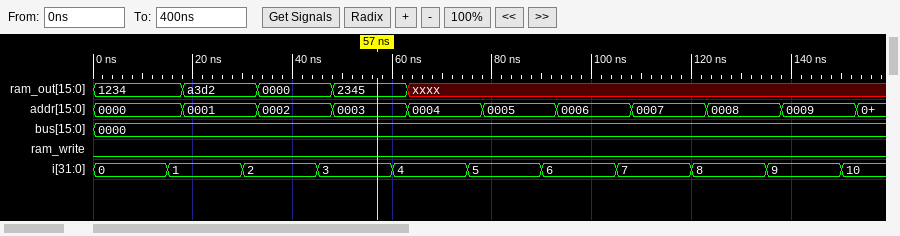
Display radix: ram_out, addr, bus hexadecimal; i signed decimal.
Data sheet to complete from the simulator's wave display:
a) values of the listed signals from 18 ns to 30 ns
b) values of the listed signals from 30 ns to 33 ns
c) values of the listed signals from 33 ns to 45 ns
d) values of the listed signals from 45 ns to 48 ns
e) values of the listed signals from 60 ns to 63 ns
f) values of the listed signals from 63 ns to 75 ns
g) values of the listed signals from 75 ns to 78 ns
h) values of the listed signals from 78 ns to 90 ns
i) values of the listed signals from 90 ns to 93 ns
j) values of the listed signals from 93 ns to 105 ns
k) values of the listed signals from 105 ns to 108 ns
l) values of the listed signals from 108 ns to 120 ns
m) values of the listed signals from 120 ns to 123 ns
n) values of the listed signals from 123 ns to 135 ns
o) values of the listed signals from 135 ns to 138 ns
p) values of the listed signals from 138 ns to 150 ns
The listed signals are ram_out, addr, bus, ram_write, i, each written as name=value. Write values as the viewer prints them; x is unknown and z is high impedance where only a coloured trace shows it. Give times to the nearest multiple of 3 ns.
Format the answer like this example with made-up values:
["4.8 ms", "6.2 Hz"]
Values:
["ram_out=a3d2, addr=0001, bus=0000, ram_write=0, i=1", "ram_out=a3d2, addr=0001, bus=0000, ram_write=0, i=2", "ram_out=0000, addr=0002, bus=0000, ram_write=0, i=2", "ram_out=0000, addr=0002, bus=0000, ram_write=0, i=3", "ram_out=2345, addr=0003, bus=0000, ram_write=0, i=4", "ram_out=xxxx, addr=0004, bus=0000, ram_write=0, i=4", "ram_out=xxxx, addr=0004, bus=0000, ram_write=0, i=5", "ram_out=xxxx, addr=0005, bus=0000, ram_write=0, i=5", "ram_out=xxxx, addr=0005, bus=0000, ram_write=0, i=6", "ram_out=xxxx, addr=0006, bus=0000, ram_write=0, i=6", "ram_out=xxxx, addr=0006, bus=0000, ram_write=0, i=7", "ram_out=xxxx, addr=0007, bus=0000, ram_write=0, i=7", "ram_out=xxxx, addr=0007, bus=0000, ram_write=0, i=8", "ram_out=xxxx, addr=0008, bus=0000, ram_write=0, i=8", "ram_out=xxxx, addr=0008, bus=0000, ram_write=0, i=9", "ram_out=xxxx, addr=0009, bus=0000, ram_write=0, i=9"]
